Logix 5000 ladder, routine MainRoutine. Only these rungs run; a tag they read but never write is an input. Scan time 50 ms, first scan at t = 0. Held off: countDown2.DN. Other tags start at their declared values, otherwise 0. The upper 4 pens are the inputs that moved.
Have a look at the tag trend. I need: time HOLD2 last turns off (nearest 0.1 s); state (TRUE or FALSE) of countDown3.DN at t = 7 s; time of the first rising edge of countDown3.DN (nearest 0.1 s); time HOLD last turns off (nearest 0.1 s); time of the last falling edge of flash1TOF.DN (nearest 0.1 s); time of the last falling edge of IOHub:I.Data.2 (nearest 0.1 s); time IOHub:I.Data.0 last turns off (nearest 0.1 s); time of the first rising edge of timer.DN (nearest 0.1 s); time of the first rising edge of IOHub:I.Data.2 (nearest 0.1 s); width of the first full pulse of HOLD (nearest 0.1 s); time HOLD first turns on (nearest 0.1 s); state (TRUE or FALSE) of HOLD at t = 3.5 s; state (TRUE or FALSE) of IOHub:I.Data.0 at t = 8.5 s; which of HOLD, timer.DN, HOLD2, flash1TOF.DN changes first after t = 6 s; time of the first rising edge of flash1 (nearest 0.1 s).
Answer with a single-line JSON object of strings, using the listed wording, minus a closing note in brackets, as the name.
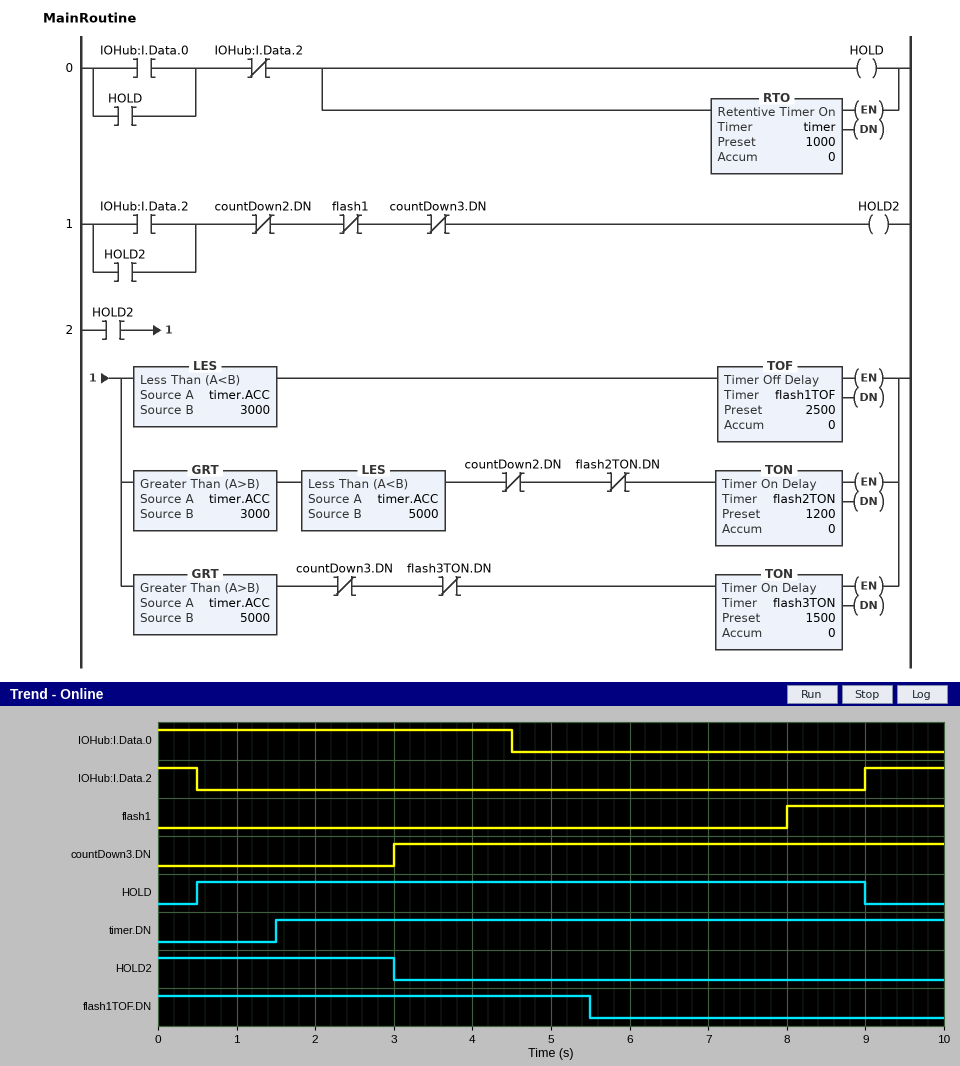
{"time HOLD2 last turns off": "3.0 s", "state (TRUE or FALSE) of countDown3.DN at t = 7 s": "TRUE", "time of the first rising edge of countDown3.DN": "3.0 s", "time HOLD last turns off": "9.0 s", "time of the last falling edge of flash1TOF.DN": "5.5 s", "time of the last falling edge of IOHub:I.Data.2": "0.5 s", "time IOHub:I.Data.0 last turns off": "4.5 s", "time of the first rising edge of timer.DN": "1.5 s", "time of the first rising edge of IOHub:I.Data.2": "9.0 s", "width of the first full pulse of HOLD": "8.5 s", "time HOLD first turns on": "0.5 s", "state (TRUE or FALSE) of HOLD at t = 3.5 s": "TRUE", "state (TRUE or FALSE) of IOHub:I.Data.0 at t = 8.5 s": "FALSE", "which of HOLD, timer.DN, HOLD2, flash1TOF.DN changes first after t = 6 s": "HOLD", "time of the first rising edge of flash1": "8.0 s"}
